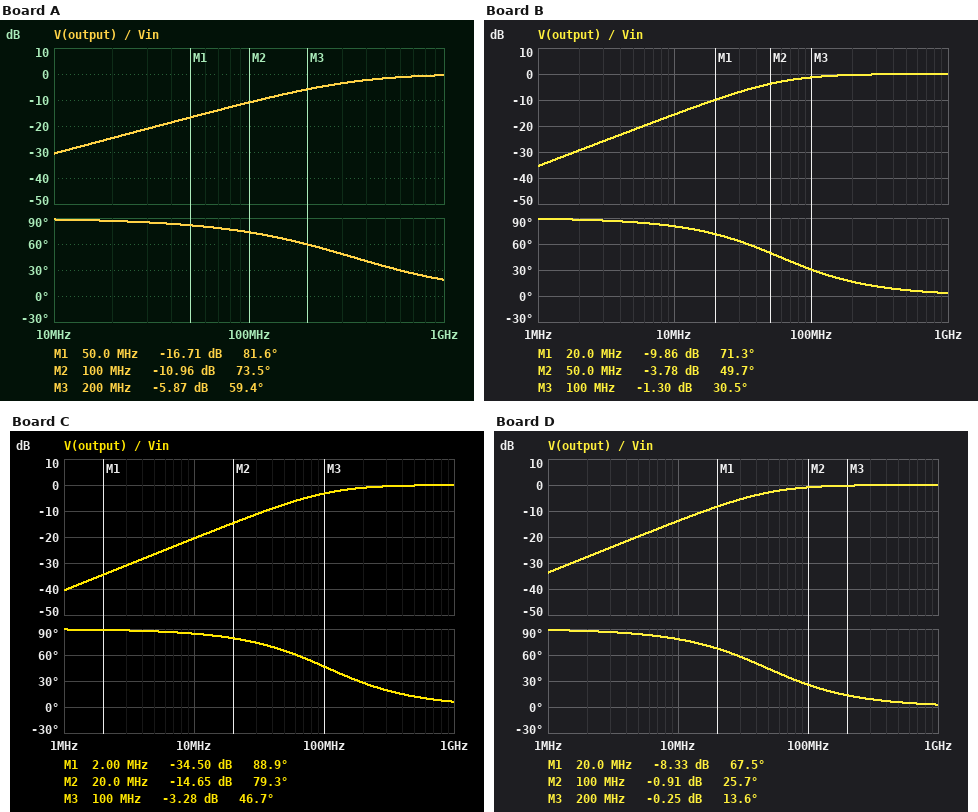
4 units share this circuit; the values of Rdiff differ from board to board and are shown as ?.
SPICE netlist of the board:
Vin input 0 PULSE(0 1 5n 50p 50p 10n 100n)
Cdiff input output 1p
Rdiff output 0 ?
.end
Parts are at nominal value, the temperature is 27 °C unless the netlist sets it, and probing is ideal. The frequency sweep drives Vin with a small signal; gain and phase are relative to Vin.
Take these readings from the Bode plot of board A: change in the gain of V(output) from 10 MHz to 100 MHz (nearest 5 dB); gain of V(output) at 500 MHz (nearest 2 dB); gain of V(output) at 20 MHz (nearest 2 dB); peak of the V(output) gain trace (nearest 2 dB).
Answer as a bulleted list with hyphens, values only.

- 20 dB
- -2 dB
- -24 dB
- 0 dB
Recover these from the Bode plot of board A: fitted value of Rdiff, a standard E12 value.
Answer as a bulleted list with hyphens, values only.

- 470 Ω
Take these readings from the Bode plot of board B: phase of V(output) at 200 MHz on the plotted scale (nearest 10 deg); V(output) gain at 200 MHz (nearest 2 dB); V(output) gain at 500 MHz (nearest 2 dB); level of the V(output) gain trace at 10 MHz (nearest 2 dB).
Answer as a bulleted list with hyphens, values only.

- 20 deg
- 0 dB
- 0 dB
- -16 dB
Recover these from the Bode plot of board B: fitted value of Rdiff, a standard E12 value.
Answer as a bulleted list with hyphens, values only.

- 2.7 kΩ
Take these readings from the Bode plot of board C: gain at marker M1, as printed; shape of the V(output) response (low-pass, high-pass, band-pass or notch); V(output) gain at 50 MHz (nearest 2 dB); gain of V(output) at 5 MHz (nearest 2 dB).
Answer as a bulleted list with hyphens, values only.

- -34.50 dB
- high-pass
- -8 dB
- -26 dB
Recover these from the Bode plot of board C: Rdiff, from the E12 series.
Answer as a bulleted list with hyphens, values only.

- 1.5 kΩ
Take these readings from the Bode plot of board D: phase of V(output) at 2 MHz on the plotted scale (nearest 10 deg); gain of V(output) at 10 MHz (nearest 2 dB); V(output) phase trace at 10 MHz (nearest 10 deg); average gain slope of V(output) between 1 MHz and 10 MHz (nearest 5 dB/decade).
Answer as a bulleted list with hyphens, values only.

- 90 deg
- -14 dB
- 80 deg
- 20 dB/decade
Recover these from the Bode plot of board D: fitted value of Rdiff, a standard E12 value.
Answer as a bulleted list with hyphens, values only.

- 3.3 kΩ
